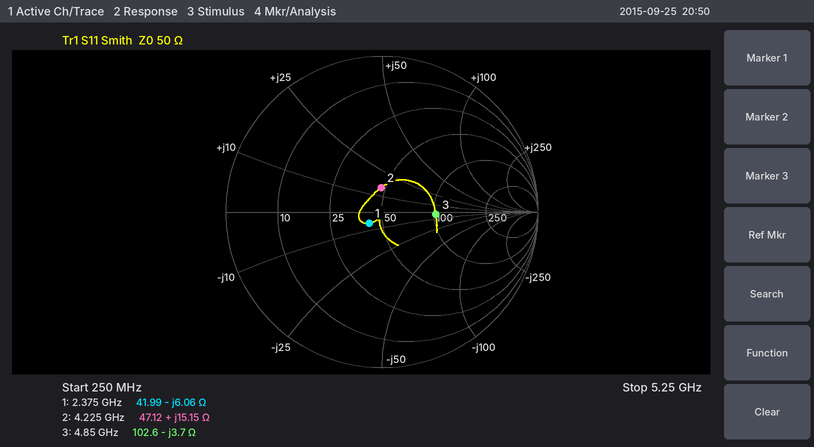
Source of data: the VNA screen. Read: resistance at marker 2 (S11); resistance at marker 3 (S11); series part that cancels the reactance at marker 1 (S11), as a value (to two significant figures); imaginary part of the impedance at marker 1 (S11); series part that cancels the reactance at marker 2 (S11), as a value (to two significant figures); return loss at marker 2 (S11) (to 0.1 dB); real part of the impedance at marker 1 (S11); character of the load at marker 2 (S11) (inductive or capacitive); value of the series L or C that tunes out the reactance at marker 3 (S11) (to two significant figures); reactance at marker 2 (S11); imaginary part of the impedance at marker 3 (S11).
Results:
47.12 Ω
102.6 Ω
410 pH
-6.06 Ω
2.5 pF
16.1 dB
41.99 Ω
inductive
120 pH
+15.15 Ω
-3.7 Ω
